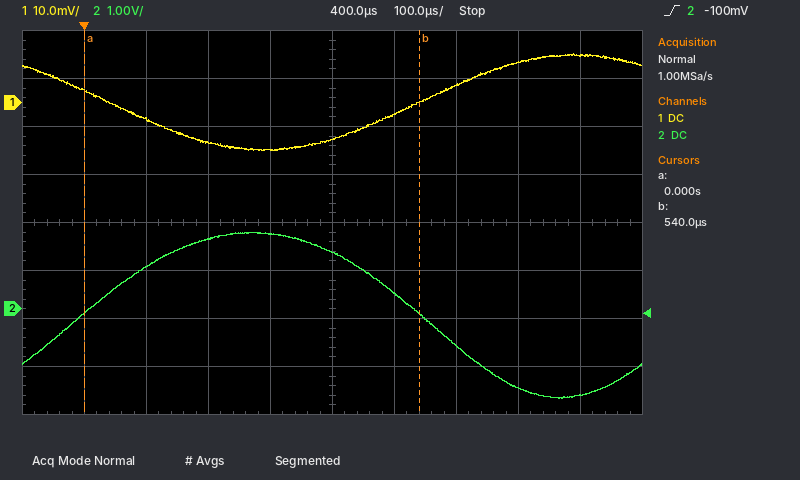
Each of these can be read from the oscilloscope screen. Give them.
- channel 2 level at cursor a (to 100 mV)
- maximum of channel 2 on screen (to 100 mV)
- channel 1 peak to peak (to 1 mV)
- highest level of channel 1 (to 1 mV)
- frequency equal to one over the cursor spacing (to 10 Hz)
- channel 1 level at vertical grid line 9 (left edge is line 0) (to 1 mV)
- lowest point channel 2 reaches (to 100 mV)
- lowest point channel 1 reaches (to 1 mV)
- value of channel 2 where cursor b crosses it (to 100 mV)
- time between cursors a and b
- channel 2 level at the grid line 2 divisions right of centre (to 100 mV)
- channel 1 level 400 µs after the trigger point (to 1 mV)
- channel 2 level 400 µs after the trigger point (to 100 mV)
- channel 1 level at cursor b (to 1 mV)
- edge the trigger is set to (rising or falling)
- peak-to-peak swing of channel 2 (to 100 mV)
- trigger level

-100 mV
1.6 V
20 mV
10 mV
1.85 kHz
10 mV
-1.9 V
-10 mV
-100 mV
540 µs
-800 mV
-8 mV
1.2 V
0 mV
rising
3.5 V
-100 mV
